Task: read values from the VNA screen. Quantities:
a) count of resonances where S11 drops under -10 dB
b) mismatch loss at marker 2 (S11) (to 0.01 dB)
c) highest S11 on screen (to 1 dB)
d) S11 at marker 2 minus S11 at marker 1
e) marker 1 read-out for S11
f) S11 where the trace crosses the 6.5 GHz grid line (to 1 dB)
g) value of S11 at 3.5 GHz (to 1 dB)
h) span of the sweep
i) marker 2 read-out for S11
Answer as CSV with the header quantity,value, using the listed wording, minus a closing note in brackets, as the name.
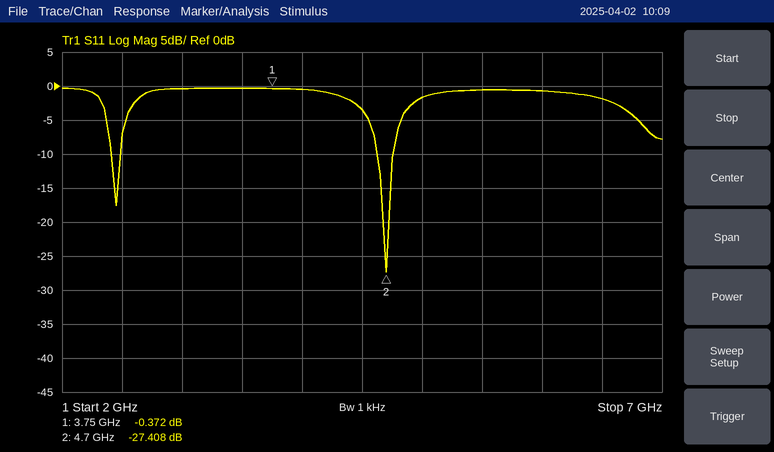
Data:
quantity,value
count of resonances where S11 drops under -10 dB,2
mismatch loss at marker 2 (S11),0.01 dB
highest S11 on screen,0 dB
S11 at marker 2 minus S11 at marker 1,-27.036 dB
marker 1 read-out for S11,-0.372 dB
S11 where the trace crosses the 6.5 GHz grid line,-2 dB
value of S11 at 3.5 GHz,0 dB
span of the sweep,5 GHz
marker 2 read-out for S11,-27.408 dB
